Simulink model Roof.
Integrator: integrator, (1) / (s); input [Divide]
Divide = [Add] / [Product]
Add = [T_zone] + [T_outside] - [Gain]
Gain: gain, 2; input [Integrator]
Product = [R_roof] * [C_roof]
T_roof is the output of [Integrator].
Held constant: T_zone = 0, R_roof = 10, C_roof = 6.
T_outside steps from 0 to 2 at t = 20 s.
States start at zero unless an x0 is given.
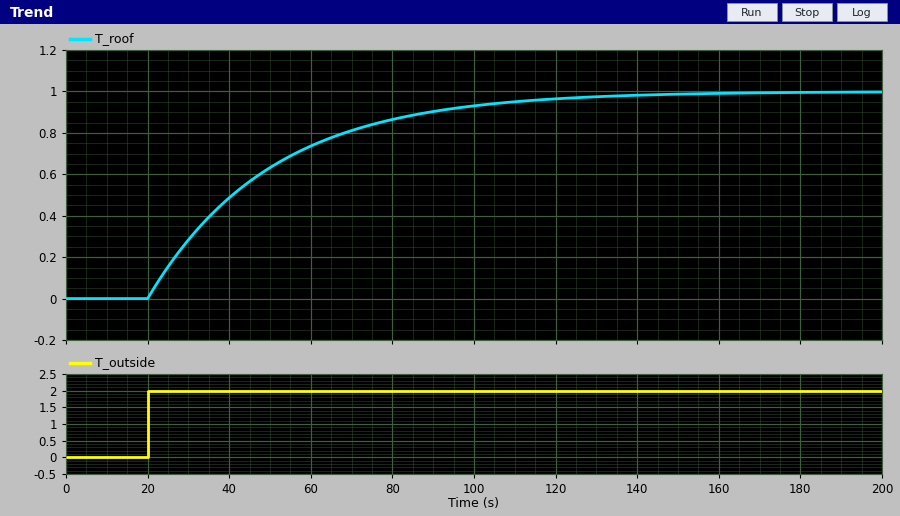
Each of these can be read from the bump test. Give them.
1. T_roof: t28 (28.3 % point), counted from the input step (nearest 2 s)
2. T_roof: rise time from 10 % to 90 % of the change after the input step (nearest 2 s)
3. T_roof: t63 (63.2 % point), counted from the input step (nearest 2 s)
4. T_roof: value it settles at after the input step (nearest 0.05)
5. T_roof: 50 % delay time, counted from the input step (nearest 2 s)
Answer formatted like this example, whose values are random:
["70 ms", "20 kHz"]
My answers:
["10 s", "66 s", "30 s", "1.00", "20 s"]
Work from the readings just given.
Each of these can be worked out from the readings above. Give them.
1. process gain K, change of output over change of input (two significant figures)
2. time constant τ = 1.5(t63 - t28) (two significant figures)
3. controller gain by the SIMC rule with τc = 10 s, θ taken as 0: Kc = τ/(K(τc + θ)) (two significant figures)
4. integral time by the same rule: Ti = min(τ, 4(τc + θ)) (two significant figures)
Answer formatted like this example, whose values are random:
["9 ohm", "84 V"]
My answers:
["0.50", "30 s", "6.0", "30 s"]
